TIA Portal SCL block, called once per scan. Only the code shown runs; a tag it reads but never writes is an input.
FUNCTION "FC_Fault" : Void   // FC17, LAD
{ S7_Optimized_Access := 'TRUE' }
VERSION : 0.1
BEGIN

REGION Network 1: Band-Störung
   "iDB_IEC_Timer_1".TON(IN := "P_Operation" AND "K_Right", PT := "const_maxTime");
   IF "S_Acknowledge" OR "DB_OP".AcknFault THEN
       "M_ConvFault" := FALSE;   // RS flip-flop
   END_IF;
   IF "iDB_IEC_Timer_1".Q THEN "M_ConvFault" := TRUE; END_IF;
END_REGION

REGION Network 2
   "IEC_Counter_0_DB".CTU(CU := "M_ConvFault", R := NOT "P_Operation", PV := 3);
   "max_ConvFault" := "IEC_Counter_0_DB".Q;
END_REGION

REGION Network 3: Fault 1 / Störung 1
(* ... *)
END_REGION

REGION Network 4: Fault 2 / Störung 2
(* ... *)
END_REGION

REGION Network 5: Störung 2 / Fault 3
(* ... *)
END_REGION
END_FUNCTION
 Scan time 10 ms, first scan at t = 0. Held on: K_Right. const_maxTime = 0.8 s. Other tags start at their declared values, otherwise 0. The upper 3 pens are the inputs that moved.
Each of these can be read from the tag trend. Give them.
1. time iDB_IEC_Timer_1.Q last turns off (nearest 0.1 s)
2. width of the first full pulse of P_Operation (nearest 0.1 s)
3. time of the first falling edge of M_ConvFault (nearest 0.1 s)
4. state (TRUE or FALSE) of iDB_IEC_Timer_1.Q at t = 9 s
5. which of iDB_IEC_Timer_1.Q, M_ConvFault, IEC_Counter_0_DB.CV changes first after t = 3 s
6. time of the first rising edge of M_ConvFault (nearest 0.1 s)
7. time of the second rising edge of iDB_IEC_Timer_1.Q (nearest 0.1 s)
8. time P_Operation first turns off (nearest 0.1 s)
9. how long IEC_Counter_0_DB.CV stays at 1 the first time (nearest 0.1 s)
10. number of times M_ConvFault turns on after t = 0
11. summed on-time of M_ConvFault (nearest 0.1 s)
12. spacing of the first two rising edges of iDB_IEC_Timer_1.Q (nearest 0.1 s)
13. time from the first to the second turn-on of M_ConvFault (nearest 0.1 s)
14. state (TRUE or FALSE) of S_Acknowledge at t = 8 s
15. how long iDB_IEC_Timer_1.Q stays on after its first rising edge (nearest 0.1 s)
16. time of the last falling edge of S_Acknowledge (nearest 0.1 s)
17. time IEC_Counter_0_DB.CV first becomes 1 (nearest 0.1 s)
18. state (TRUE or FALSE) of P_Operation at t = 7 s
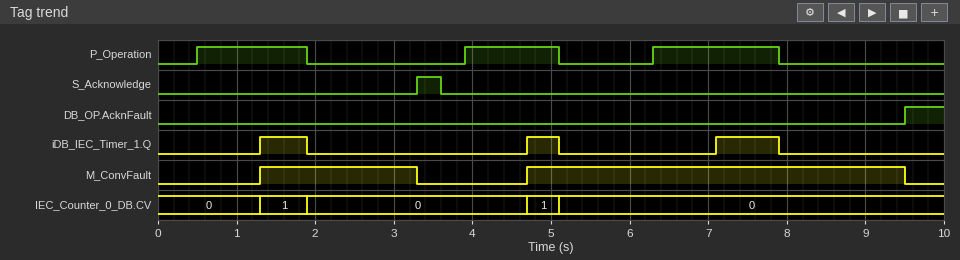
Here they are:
7.9 s
1.4 s
3.3 s
FALSE
M_ConvFault
1.3 s
4.7 s
1.9 s
0.6 s
2
6.8 s
3.4 s
3.4 s
FALSE
0.6 s
3.6 s
1.3 s
TRUE
